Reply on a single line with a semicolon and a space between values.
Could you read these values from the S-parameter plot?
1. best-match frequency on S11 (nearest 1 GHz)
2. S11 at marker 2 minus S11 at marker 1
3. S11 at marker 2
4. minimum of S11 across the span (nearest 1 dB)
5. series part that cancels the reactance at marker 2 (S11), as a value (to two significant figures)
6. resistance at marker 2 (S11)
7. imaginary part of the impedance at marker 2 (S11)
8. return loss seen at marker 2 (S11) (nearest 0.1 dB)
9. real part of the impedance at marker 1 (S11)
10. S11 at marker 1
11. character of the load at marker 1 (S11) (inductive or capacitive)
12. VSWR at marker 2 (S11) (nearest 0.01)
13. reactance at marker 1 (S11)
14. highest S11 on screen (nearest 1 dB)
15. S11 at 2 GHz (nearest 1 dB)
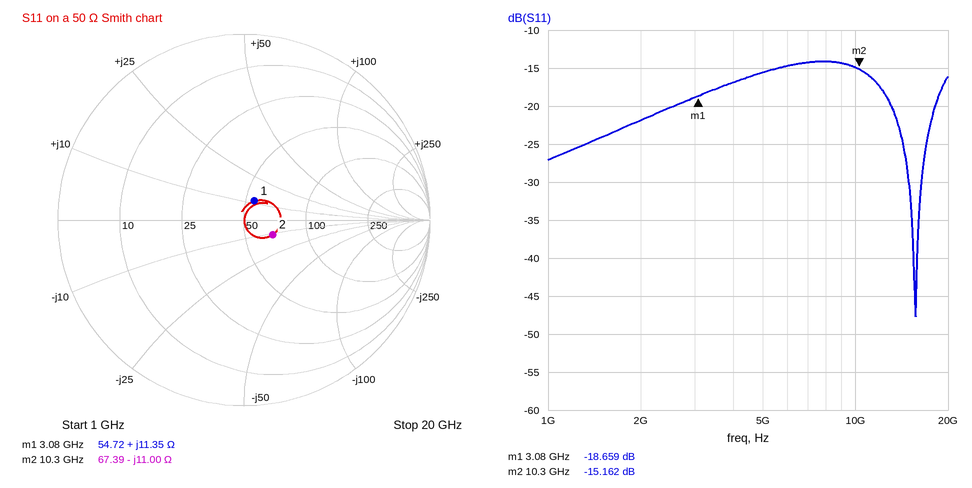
16 GHz; 3.497 dB; -15.162 dB; -48 dB; 170 pH; 67.39 Ω; -11.00 Ω; 15.2 dB; 54.72 Ω; -18.659 dB; inductive; 1.42; +11.35 Ω; -14 dB; -22 dB
